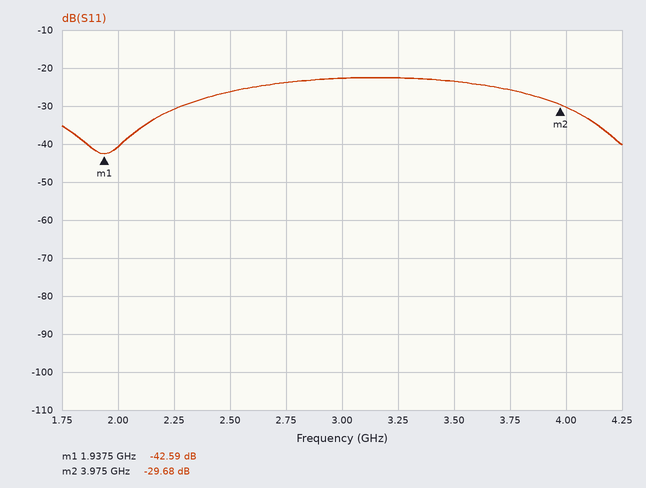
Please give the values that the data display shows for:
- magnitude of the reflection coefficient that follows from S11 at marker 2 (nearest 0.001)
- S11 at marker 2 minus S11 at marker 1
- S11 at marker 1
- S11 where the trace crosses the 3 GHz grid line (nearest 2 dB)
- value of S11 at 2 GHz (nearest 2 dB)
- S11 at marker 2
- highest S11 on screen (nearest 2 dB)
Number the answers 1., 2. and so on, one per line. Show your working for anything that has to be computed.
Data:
1. 10^(-29.68/20) ≈ 0.033
2. -29.68 − (-42.59) = 12.91 dB
3. -42.59 dB
4. -22 dB
5. -40 dB
6. -29.68 dB
7. -22 dB
